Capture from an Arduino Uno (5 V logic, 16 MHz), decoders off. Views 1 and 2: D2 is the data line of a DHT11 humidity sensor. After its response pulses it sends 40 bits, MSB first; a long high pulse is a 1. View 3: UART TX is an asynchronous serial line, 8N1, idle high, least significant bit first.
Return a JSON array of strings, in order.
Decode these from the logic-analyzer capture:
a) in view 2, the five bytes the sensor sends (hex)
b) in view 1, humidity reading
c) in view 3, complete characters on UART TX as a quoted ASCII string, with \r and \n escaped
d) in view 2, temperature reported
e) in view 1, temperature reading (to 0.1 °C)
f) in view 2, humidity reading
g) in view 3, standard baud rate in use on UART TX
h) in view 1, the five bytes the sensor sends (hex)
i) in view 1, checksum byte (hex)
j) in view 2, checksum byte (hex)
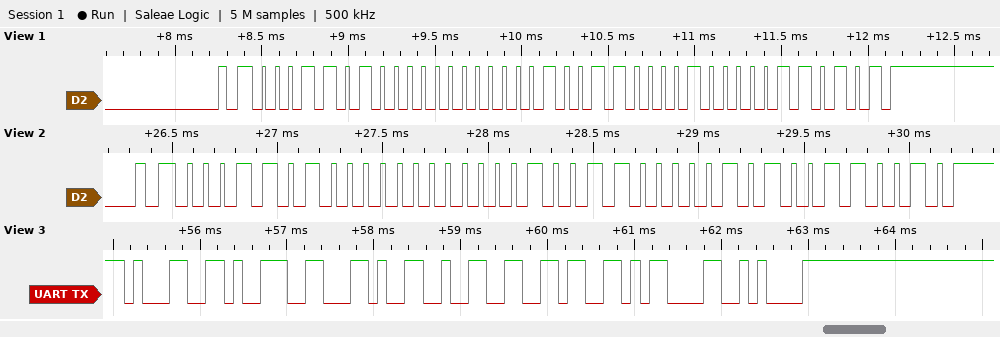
["1A 00 13 05 32", "26 %", "\"19,26\\r\\n\"", "19.5 °C", "19.8 °C", "26 %", "9600 baud", "1A 00 13 08 35", "0x35", "0x32"]
